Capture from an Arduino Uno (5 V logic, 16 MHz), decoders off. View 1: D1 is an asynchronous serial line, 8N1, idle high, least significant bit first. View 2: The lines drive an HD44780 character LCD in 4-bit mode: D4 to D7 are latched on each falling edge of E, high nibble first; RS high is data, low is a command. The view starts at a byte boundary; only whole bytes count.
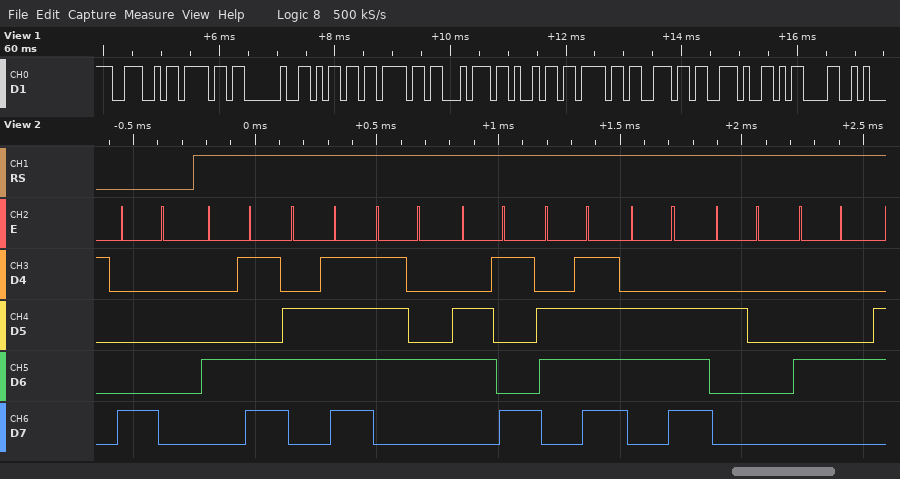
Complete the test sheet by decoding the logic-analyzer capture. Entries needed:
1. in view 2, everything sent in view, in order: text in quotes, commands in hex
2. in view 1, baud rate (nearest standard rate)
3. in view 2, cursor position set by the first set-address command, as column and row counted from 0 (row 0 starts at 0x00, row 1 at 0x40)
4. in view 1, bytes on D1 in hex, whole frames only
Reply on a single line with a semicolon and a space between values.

0x80 "Motion D"; 9600 baud; column 0, row 0; 0x4E 0x6F 0x20 0x6D 0x6F 0x74 0x69 0x6F 0x6E 0x2E 0x0D
